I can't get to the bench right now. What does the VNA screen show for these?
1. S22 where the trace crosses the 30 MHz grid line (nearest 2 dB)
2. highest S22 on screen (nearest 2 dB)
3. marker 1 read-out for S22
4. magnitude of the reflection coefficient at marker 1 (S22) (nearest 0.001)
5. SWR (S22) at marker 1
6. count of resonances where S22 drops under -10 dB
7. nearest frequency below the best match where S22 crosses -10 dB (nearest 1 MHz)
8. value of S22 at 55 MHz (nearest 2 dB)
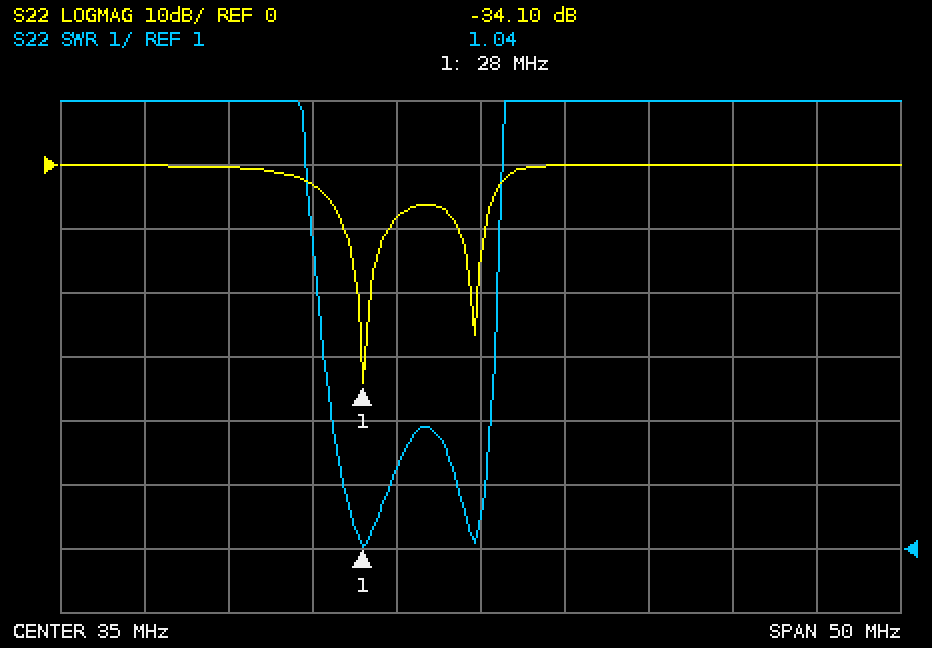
-8 dB
0 dB
-34.10 dB
0.020
1.04
2
27 MHz
0 dB
